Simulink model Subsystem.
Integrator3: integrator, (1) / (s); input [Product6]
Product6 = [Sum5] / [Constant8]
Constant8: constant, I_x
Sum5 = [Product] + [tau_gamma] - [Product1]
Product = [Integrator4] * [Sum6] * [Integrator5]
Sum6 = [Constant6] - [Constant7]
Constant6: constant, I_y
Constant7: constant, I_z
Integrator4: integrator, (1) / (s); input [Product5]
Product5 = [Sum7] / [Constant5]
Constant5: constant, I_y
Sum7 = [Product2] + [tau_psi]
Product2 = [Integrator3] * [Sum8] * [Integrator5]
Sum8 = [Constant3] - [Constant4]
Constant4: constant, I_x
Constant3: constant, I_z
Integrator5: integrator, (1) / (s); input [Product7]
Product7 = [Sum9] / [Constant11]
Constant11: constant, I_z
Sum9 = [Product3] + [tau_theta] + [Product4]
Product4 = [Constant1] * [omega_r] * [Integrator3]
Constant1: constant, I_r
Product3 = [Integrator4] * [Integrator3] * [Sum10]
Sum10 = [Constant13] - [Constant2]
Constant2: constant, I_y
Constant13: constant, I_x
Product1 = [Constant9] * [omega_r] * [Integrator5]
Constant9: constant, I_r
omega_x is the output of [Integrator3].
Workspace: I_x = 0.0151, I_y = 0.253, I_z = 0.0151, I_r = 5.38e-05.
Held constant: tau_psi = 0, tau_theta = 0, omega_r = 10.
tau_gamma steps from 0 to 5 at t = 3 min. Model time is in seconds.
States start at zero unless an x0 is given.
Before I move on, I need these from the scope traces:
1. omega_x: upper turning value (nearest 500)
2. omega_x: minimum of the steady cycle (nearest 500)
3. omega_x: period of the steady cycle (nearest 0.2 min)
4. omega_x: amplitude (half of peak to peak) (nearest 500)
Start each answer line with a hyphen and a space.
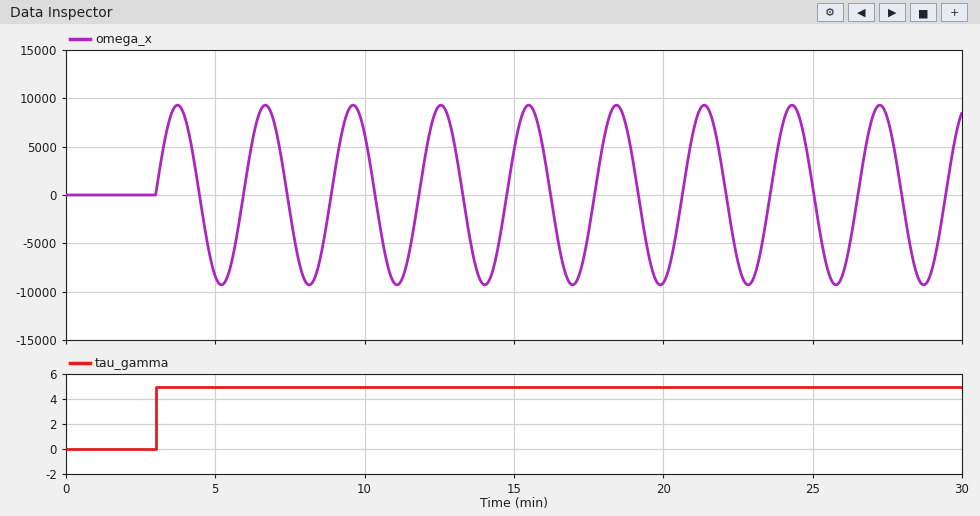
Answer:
- 9500
- -9500
- 3.0 min
- 9500
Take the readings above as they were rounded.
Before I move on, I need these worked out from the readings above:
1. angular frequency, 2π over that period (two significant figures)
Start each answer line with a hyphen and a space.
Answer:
- 2.1 rad/min
